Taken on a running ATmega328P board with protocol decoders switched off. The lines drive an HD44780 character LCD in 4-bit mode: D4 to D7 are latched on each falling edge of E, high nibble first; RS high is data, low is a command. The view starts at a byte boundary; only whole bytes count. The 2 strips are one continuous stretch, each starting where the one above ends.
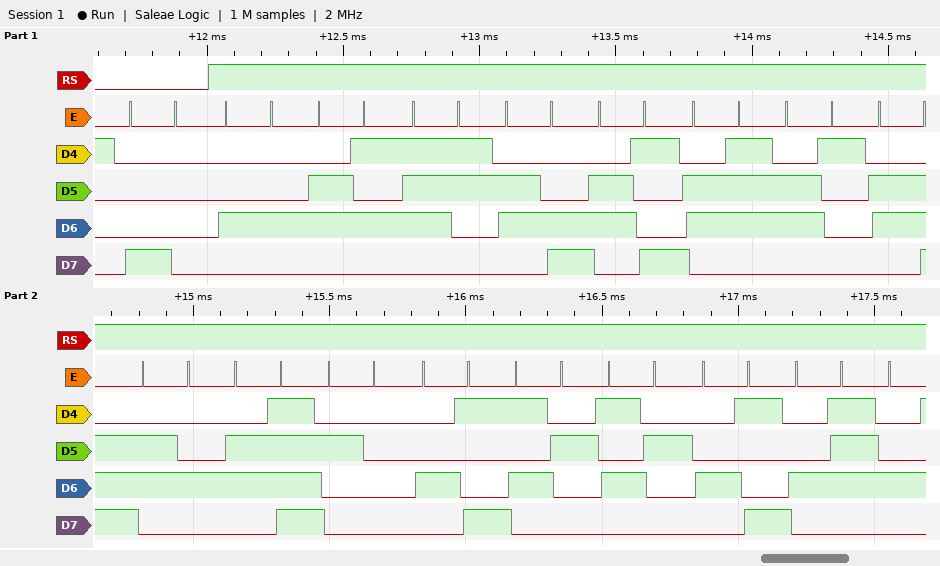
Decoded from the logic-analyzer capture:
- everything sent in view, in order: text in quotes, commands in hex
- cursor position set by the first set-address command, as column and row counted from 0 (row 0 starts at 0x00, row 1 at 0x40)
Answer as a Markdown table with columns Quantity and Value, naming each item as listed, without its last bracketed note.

| Quantity | Value |
|---|---|
| everything sent in view, in order: text in quotes, commands in hex | 0x80 "Desligando IRRIG" |
| cursor position set by the first set-address command, as column and row counted from 0 | column 0, row 0 |
